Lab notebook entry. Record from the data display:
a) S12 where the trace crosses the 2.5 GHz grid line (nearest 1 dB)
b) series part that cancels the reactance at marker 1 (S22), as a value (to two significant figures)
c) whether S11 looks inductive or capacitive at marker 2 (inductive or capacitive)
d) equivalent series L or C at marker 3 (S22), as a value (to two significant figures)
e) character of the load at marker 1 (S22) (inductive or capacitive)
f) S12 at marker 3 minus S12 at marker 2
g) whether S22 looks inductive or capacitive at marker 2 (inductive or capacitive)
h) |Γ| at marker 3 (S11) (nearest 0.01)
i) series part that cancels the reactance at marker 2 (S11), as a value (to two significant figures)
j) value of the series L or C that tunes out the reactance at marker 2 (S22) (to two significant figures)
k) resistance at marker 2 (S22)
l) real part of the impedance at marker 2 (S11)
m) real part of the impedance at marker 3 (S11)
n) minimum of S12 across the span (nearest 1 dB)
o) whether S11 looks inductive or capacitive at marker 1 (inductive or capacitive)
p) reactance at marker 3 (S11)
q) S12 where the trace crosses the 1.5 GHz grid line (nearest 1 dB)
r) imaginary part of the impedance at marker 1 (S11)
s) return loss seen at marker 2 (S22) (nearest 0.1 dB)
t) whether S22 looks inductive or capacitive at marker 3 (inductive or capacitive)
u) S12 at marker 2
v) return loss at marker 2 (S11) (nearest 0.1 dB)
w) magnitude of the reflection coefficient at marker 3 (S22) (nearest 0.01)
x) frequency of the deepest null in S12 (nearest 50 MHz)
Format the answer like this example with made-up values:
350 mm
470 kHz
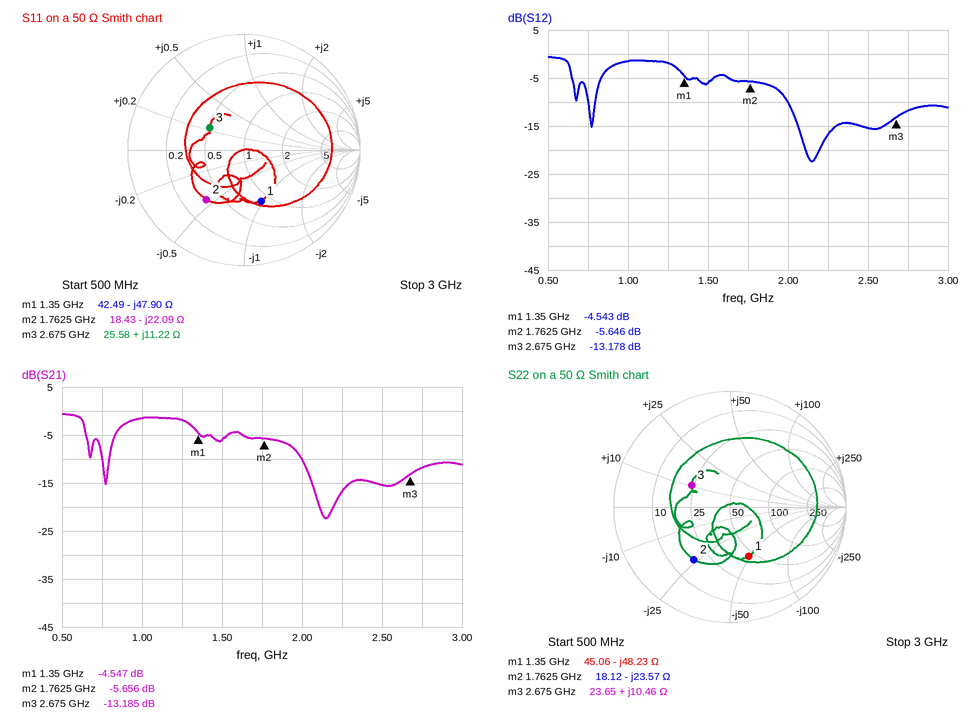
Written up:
-15 dB
5.7 nH
capacitive
620 pH
capacitive
-7.532 dB
capacitive
0.35
2.0 nH
2.1 nH
18.12 Ω
18.43 Ω
25.58 Ω
-22 dB
capacitive
+11.22 Ω
-6 dB
-47.90 Ω
5.2 dB
inductive
-5.646 dB
5.4 dB
0.38
2.15 GHz
